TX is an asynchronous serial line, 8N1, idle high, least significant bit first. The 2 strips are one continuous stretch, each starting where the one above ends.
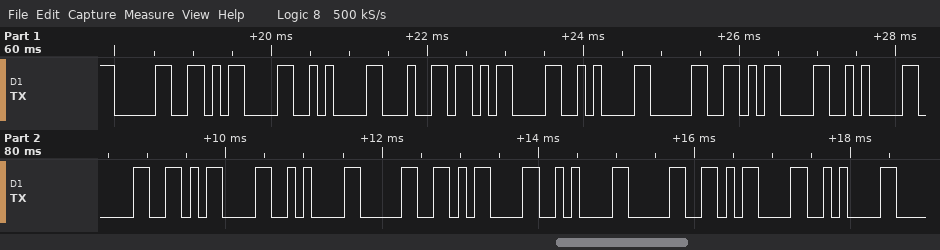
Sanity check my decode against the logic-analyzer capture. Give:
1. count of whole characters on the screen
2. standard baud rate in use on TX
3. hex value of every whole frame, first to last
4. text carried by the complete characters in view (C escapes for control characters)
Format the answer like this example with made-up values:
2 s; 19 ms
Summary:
18; 9600 baud; 30 0D 0A 64 0D 0A 30 0D 0A 30 0D 0A 30 0D 0A 30 0D 0A; "0\r\nd\r\n0\r\n0\r\n0\r\n0\r\n"
